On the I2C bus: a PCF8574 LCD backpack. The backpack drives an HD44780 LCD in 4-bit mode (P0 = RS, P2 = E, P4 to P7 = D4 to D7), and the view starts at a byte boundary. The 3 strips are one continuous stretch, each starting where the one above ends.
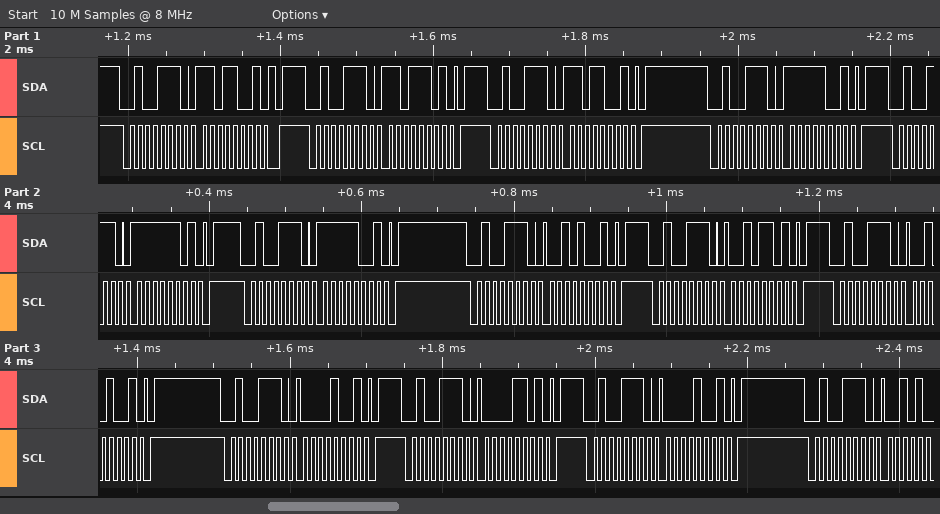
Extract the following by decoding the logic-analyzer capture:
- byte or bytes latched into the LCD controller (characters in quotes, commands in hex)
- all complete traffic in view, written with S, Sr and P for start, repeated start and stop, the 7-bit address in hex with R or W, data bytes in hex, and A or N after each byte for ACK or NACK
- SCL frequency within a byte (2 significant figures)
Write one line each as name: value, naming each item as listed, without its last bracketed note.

byte or bytes latched into the LCD controller: data 0xDF ' '
all complete traffic in view, written with S, Sr and P for start, repeated start and stop, the 7-bit address in hex with R or W, data bytes in hex, and A or N after each byte for ACK or NACK: S 27W A D9 A P S 27W A DD A P S 27W A D9 A P S 27W A F9 A P S 27W A FD A P S 27W A F9 A P S 27W A 29 A P S 27W A 2D A P S 27W A 29 A P S 27W A 09 A P S 27W A 0D A P S 27W A 09 A P S 27W A
SCL frequency within a byte: 100 kHz
